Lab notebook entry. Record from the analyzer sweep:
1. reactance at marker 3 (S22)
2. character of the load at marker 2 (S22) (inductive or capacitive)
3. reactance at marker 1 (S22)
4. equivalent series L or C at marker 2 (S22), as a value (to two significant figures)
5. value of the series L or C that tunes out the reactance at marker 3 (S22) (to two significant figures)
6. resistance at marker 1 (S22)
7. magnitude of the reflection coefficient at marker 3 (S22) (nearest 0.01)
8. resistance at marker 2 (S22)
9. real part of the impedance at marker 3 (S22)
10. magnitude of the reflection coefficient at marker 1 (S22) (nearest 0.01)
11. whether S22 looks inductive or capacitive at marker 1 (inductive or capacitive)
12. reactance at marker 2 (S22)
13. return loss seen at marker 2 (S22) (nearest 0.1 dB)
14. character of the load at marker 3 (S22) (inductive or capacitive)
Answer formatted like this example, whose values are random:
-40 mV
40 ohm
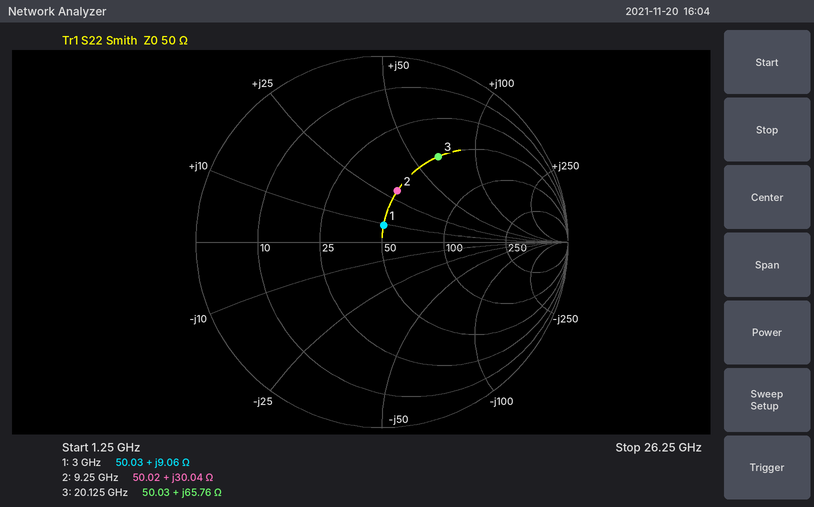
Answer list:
+65.76 Ω
inductive
+9.06 Ω
520 pH
120 fF
50.03 Ω
0.55
50.02 Ω
50.03 Ω
0.09
inductive
+30.04 Ω
10.8 dB
inductive
